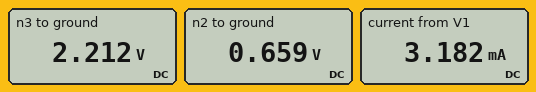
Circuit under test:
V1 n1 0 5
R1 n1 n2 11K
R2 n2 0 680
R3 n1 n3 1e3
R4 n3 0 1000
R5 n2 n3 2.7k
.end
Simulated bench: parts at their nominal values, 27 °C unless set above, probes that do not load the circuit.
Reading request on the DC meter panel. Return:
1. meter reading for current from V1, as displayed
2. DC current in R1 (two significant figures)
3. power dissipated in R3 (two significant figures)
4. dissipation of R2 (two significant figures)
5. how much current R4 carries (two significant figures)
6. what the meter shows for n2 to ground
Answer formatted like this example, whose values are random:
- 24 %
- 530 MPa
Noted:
- 3.182 mA
- 390 µA
- 7.8 mW
- 640 µW
- 2.2 mA
- 0.659 V
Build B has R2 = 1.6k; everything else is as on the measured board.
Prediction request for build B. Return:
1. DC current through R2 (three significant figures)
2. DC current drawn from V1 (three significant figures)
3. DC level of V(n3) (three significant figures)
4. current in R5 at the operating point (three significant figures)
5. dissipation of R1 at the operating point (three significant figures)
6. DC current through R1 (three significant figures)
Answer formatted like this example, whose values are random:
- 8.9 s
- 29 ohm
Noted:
- 751 µA
- 3.05 mA
- 2.30 V
- 406 µA
- 1.31 mW
- 345 µA
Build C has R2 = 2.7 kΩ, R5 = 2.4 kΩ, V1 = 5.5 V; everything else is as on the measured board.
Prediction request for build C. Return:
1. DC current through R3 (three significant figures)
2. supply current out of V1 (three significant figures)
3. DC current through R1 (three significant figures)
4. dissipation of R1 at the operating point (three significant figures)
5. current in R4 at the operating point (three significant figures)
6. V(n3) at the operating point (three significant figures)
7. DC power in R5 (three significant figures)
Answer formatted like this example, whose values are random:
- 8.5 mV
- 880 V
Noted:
- 2.91 mA
- 3.25 mA
- 337 µA
- 1.25 mW
- 2.59 mA
- 2.59 V
- 259 µW
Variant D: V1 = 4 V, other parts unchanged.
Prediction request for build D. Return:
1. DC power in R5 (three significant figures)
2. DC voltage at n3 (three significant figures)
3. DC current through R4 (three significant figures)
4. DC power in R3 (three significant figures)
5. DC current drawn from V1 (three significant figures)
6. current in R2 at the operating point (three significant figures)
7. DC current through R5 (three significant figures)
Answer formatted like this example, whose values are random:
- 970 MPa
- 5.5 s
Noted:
- 572 µW
- 1.77 V
- 1.77 mA
- 4.97 mW
- 2.55 mA
- 776 µA
- 460 µA
